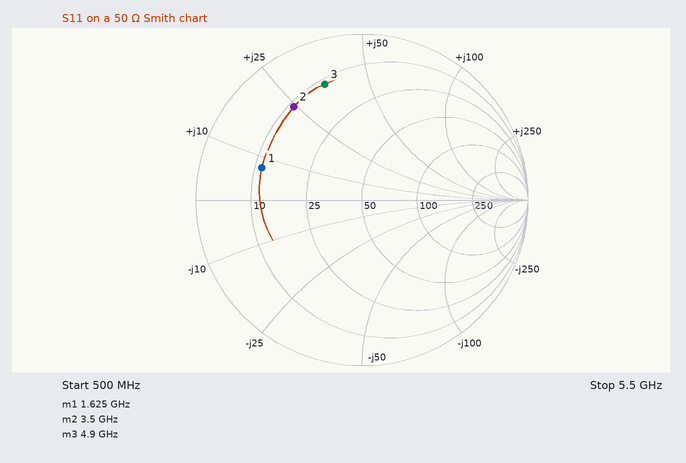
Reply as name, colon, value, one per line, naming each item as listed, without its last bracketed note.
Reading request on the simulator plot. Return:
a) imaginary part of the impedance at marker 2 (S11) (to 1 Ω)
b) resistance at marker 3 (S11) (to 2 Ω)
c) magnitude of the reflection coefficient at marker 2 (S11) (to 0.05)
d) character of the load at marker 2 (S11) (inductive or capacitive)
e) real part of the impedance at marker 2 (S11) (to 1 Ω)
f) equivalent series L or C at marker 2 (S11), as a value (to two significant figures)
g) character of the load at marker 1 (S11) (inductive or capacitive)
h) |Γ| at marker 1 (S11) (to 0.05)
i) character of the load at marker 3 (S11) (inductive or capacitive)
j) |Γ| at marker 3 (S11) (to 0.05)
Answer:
imaginary part of the impedance at marker 2 (S11): +24 Ω
resistance at marker 3 (S11): 12 Ω
magnitude of the reflection coefficient at marker 2 (S11): 0.70
character of the load at marker 2 (S11): inductive
real part of the impedance at marker 2 (S11): 11 Ω
equivalent series L or C at marker 2 (S11), as a value: 1.1 nH
character of the load at marker 1 (S11): inductive
|Γ| at marker 1 (S11): 0.65
character of the load at marker 3 (S11): inductive
|Γ| at marker 3 (S11): 0.75
